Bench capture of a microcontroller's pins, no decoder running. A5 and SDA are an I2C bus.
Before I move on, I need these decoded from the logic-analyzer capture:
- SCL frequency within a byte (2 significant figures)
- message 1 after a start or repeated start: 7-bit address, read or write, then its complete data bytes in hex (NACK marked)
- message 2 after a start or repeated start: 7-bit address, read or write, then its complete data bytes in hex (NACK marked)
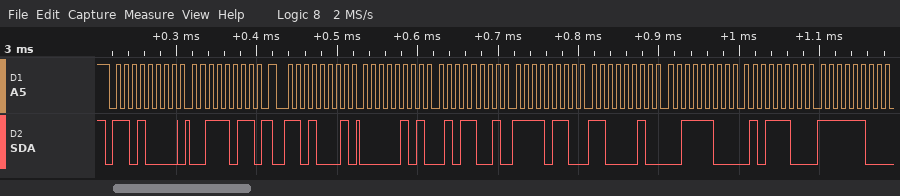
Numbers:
100 kHz
0x68 write: 3B
0x68 read: 05 59 F6 C2 3C 5C FC
